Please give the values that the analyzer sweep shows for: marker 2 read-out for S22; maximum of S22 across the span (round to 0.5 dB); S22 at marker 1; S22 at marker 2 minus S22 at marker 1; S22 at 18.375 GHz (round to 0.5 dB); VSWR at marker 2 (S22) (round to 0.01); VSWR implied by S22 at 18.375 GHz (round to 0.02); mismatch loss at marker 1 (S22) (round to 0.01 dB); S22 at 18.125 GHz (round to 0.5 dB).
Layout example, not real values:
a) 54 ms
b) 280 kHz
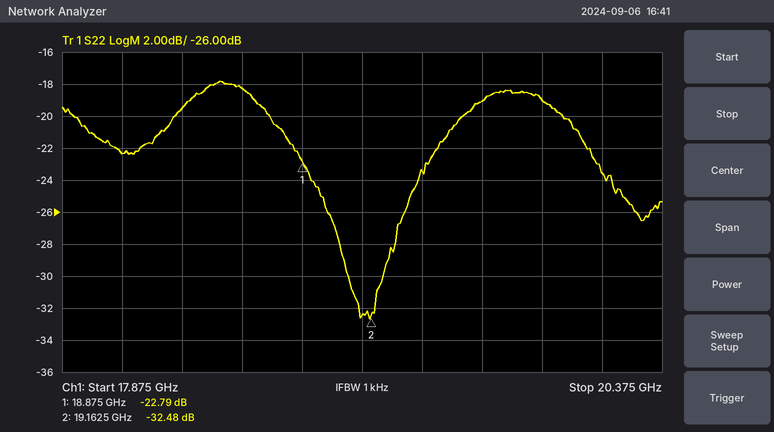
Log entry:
a) -32.48 dB
b) -18.0 dB
c) -22.79 dB
d) -9.69 dB
e) -19.5 dB
f) 1.05
g) 1.24
h) 0.02 dB
i) -22.5 dB
